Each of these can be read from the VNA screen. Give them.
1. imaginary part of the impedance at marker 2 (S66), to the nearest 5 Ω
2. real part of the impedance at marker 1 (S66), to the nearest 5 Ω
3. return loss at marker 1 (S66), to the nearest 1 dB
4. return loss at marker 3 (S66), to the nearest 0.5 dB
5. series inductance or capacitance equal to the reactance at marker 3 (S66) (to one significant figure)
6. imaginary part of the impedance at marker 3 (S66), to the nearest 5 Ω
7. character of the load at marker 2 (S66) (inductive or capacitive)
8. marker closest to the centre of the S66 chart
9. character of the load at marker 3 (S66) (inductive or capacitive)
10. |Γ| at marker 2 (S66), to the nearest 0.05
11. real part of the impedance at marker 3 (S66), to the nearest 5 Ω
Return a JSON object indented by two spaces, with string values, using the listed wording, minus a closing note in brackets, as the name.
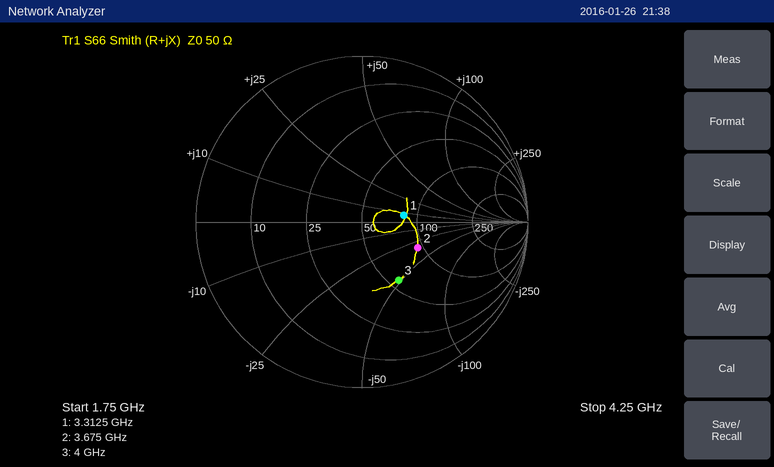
{
  "imaginary part of the impedance at marker 2 (S66), to the nearest 5 Ω": "-35 Ω",
  "real part of the impedance at marker 1 (S66), to the nearest 5 Ω": "85 Ω",
  "return loss at marker 1 (S66), to the nearest 1 dB": "12 dB",
  "return loss at marker 3 (S66), to the nearest 0.5 dB": "7.5 dB",
  "series inductance or capacitance equal to the reactance at marker 3 (S66)": "800 fF",
  "imaginary part of the impedance at marker 3 (S66), to the nearest 5 Ω": "-50 Ω",
  "character of the load at marker 2 (S66)": "capacitive",
  "marker closest to the centre of the S66 chart": "marker 1",
  "character of the load at marker 3 (S66)": "capacitive",
  "|Γ| at marker 2 (S66), to the nearest 0.05": "0.35",
  "real part of the impedance at marker 3 (S66), to the nearest 5 Ω": "55 Ω"
}
